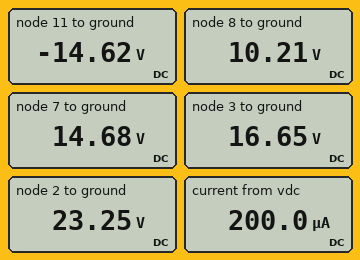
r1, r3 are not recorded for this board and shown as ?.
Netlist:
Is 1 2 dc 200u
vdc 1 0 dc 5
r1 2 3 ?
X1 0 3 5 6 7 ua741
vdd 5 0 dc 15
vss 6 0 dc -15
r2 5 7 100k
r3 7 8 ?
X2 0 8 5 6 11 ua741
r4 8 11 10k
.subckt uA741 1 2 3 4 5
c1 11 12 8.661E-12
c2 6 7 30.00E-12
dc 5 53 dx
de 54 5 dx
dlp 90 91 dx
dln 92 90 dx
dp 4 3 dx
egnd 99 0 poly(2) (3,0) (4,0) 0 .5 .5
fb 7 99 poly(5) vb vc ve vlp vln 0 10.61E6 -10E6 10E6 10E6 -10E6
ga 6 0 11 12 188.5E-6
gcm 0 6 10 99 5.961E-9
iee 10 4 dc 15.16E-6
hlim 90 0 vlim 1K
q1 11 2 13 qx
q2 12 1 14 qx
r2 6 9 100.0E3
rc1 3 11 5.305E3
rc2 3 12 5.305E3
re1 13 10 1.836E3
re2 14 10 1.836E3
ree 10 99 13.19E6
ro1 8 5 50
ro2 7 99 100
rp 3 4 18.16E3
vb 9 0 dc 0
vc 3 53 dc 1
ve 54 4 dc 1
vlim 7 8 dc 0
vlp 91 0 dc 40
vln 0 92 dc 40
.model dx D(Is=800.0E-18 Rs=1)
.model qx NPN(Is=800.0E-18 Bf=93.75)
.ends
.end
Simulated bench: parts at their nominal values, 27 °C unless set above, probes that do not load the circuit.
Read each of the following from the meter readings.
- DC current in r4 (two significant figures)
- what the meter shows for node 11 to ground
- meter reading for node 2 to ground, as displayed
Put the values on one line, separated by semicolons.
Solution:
2.5 mA; -14.62 V; 23.25 V
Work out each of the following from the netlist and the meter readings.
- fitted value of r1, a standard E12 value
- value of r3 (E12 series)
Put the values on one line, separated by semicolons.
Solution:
33 kΩ; 1.8 kΩ
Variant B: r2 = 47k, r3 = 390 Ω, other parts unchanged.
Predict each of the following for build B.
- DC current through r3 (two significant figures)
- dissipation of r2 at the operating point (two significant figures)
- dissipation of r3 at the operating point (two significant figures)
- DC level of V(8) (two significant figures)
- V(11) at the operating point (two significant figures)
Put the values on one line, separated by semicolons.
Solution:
2.8 mA; 2.2 µW; 3.1 mW; 14 V; -15 V
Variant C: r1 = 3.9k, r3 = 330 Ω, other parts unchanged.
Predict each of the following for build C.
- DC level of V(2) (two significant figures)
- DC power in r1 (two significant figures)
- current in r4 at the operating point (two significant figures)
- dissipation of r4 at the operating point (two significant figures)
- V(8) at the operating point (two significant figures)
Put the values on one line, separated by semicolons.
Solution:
17 V; 160 µW; 2.8 mA; 80 mW; 14 V
